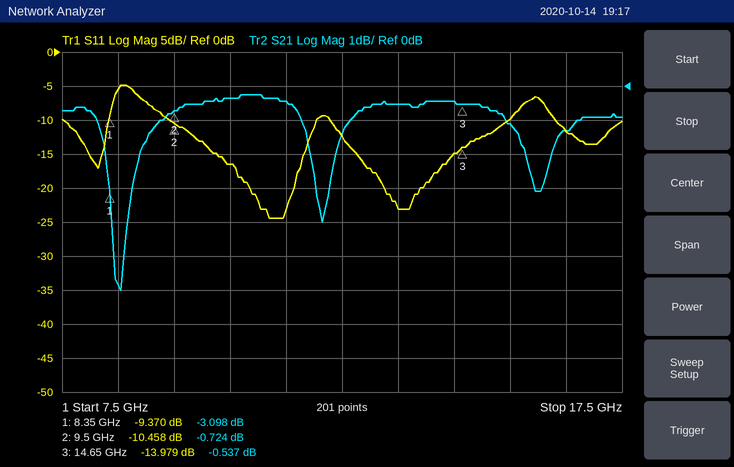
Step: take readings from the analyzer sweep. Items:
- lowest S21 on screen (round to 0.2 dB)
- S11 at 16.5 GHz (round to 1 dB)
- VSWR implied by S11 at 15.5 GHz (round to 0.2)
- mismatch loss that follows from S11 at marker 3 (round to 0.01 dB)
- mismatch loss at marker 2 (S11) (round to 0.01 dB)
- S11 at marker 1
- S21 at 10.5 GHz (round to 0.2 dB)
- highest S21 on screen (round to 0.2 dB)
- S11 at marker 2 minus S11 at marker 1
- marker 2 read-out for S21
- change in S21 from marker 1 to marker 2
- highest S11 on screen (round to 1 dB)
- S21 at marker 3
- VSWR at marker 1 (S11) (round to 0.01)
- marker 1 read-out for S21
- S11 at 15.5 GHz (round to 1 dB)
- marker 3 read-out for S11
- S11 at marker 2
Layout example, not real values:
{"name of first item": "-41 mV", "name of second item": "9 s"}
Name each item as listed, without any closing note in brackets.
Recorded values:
{"lowest S21 on screen": "-6.0 dB", "S11 at 16.5 GHz": "-12 dB", "VSWR implied by S11 at 15.5 GHz": "2.0", "mismatch loss that follows from S11 at marker 3": "0.18 dB", "mismatch loss at marker 2 (S11)": "0.41 dB", "S11 at marker 1": "-9.370 dB", "S21 at 10.5 GHz": "-0.4 dB", "highest S21 on screen": "-0.2 dB", "S11 at marker 2 minus S11 at marker 1": "-1.088 dB", "marker 2 read-out for S21": "-0.724 dB", "change in S21 from marker 1 to marker 2": "2.374 dB", "highest S11 on screen": "-5 dB", "S21 at marker 3": "-0.537 dB", "VSWR at marker 1 (S11)": "2.03", "marker 1 read-out for S21": "-3.098 dB", "S11 at 15.5 GHz": "-10 dB", "marker 3 read-out for S11": "-13.979 dB", "S11 at marker 2": "-10.458 dB"}
